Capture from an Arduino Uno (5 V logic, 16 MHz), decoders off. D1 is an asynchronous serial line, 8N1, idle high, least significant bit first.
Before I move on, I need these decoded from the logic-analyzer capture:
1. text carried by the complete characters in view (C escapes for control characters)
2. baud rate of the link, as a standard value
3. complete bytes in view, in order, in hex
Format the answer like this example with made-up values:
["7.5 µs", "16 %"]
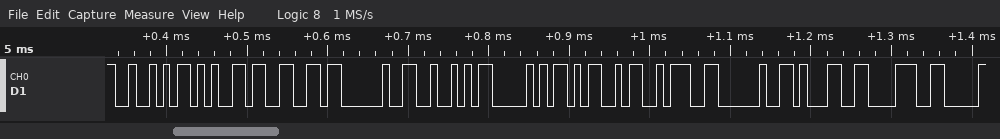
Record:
["\"Ref RPM: 18\"", "115200 baud", "0x52 0x65 0x66 0x20 0x52 0x50 0x4D 0x3A 0x20 0x31 0x38"]
